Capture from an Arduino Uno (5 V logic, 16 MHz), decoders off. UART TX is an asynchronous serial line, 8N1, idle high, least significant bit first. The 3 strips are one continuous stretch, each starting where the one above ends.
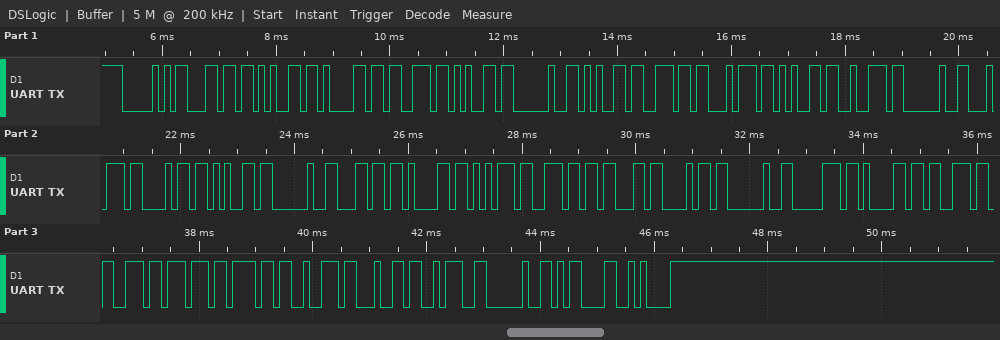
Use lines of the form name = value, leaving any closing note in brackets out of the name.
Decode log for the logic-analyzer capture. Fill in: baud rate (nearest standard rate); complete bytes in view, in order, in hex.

baud rate = 9600 baud
complete bytes in view, in order, in hex = 50 6C 65 61 73 65 20 65 6E 74 65 72 20 74 68 65 20 6C 61 75 6E 63 68 20 70 61 73 73 77 6F 72 64 3A 20 0D 0A
